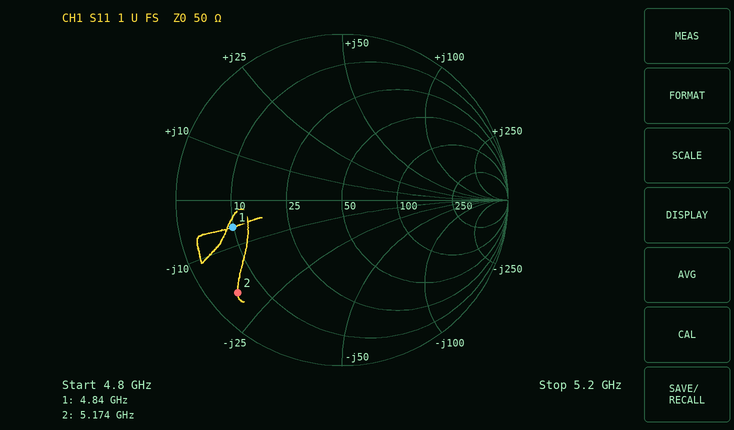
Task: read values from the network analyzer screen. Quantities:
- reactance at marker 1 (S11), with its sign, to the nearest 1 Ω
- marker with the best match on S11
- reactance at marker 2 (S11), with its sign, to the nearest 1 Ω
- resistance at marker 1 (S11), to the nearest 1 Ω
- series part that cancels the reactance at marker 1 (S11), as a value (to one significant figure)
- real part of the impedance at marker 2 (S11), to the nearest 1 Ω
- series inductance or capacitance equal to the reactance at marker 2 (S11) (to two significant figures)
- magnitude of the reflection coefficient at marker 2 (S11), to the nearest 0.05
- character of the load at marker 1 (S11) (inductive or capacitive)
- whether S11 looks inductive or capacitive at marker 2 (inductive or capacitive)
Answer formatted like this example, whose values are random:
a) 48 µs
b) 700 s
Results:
a) -6 Ω
b) marker 1
c) -19 Ω
d) 10 Ω
e) 200 pH
f) 5 Ω
g) 1.6 pF
h) 0.85
i) capacitive
j) capacitive
